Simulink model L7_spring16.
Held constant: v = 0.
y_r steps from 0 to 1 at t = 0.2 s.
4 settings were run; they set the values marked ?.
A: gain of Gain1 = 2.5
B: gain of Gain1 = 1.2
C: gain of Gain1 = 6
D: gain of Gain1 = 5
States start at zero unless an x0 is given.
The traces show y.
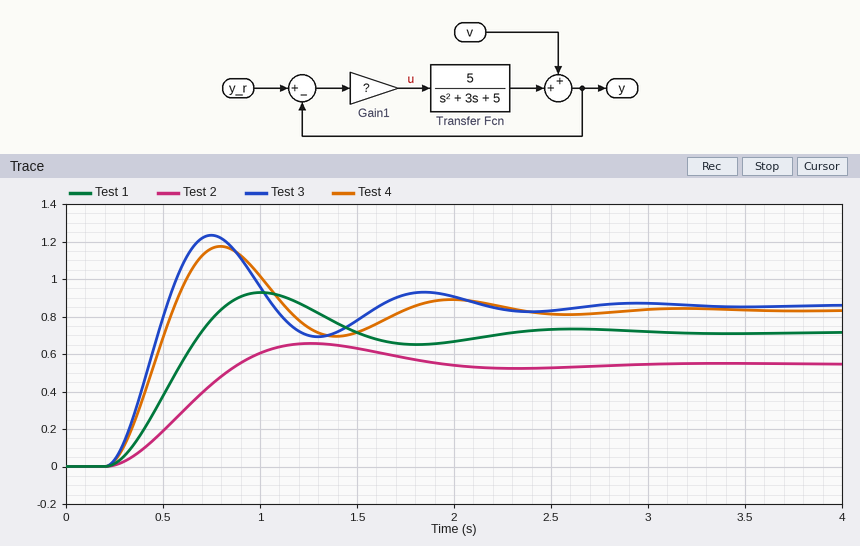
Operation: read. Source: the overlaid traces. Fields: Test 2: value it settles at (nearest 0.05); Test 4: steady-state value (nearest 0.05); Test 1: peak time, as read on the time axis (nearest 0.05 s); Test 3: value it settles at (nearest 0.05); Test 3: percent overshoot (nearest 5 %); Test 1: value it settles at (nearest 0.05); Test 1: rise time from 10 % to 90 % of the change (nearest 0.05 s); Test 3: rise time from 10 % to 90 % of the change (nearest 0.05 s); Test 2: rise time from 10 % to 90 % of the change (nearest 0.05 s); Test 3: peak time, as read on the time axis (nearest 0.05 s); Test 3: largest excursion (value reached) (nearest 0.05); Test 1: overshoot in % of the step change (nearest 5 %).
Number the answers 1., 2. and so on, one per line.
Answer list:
1. 0.55
2. 0.85
3. 1.00 s
4. 0.85
5. 45 %
6. 0.70
7. 0.35 s
8. 0.20 s
9. 0.45 s
10. 0.75 s
11. 1.25
12. 30 %
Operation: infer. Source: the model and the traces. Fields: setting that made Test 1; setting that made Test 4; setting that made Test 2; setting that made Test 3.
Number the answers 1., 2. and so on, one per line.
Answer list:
1. A
2. D
3. B
4. C
